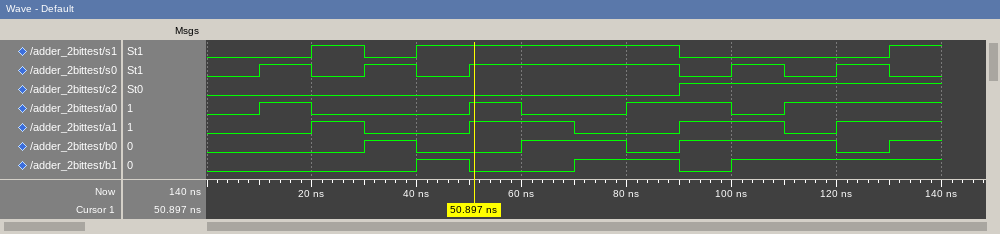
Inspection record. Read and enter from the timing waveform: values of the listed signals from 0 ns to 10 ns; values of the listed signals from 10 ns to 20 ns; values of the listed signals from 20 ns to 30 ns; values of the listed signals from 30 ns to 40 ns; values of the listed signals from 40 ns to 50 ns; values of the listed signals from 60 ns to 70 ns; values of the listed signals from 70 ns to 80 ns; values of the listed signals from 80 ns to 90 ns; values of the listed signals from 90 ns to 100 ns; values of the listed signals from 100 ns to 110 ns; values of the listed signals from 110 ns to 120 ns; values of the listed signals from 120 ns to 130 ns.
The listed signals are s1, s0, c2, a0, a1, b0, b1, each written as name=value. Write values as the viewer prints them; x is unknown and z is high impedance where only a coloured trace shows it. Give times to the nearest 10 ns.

s1=0, s0=0, c2=0, a0=0, a1=0, b0=0, b1=0
s1=0, s0=1, c2=0, a0=1, a1=0, b0=0, b1=0
s1=1, s0=0, c2=0, a0=0, a1=1, b0=0, b1=0
s1=0, s0=1, c2=0, a0=0, a1=0, b0=1, b1=0
s1=1, s0=0, c2=0, a0=0, a1=0, b0=0, b1=1
s1=1, s0=1, c2=0, a0=0, a1=1, b0=1, b1=0
s1=1, s0=1, c2=0, a0=0, a1=0, b0=1, b1=1
s1=1, s0=1, c2=0, a0=1, a1=0, b0=0, b1=1
s1=0, s0=0, c2=1, a0=1, a1=1, b0=1, b1=0
s1=0, s0=1, c2=1, a0=0, a1=1, b0=1, b1=1
s1=0, s0=0, c2=1, a0=1, a1=0, b0=1, b1=1
s1=0, s0=1, c2=1, a0=1, a1=1, b0=0, b1=1
